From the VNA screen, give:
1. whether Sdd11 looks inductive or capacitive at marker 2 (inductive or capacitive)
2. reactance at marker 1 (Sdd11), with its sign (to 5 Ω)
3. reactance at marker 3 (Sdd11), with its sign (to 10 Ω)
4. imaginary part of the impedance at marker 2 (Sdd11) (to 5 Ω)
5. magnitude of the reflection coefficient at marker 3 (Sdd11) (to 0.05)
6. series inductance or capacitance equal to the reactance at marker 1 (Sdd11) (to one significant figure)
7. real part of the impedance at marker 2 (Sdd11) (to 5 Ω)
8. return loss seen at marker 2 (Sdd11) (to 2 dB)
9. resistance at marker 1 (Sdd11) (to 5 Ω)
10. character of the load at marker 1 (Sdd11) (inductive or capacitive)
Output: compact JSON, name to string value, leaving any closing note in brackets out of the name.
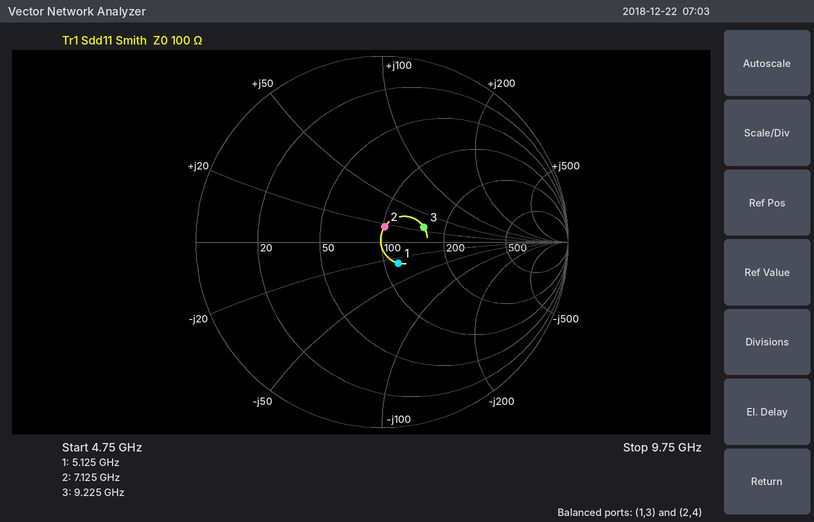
{"whether Sdd11 looks inductive or capacitive at marker 2": "inductive", "reactance at marker 1 (Sdd11), with its sign": "-25 Ω", "reactance at marker 3 (Sdd11), with its sign": "+30 Ω", "imaginary part of the impedance at marker 2 (Sdd11)": "+15 Ω", "magnitude of the reflection coefficient at marker 3 (Sdd11)": "0.25", "series inductance or capacitance equal to the reactance at marker 1 (Sdd11)": "1 pF", "real part of the impedance at marker 2 (Sdd11)": "100 Ω", "return loss seen at marker 2 (Sdd11)": "22 dB", "resistance at marker 1 (Sdd11)": "115 Ω", "character of the load at marker 1 (Sdd11)": "capacitive"}
